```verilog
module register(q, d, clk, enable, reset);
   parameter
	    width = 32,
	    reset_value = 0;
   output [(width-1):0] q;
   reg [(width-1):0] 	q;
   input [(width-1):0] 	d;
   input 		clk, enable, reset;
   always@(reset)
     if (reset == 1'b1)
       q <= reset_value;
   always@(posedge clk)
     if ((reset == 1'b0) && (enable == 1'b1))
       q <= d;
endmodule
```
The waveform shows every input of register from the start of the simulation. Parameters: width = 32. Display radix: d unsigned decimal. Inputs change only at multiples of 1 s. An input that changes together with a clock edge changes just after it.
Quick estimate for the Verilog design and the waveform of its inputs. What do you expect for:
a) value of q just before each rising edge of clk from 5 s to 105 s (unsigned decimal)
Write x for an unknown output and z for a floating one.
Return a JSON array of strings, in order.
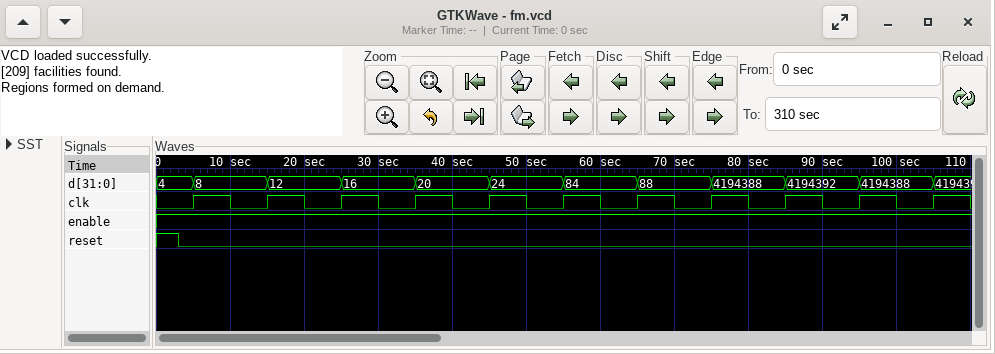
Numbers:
["0, 4, 8, 12, 16, 20, 24, 84, 88, 4194388, 4194392"]
